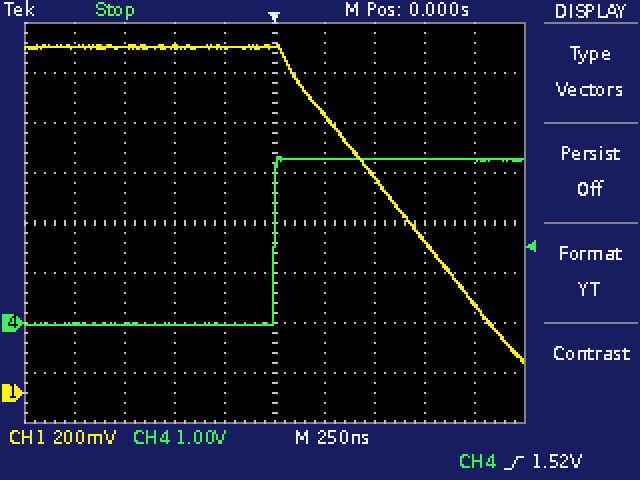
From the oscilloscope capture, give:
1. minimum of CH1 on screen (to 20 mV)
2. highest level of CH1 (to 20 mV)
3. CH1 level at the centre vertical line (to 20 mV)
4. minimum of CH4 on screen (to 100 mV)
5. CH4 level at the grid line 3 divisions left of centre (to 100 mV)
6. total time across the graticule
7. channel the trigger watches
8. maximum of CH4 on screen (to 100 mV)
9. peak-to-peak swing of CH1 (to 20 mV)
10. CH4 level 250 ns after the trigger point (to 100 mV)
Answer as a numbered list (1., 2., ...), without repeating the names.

1. 120 mV
2. 1.40 V
3. 1.38 V
4. 0.0 V
5. 0.0 V
6. 2.5 µs
7. CH4
8. 3.3 V
9. 1.28 V
10. 3.3 V
